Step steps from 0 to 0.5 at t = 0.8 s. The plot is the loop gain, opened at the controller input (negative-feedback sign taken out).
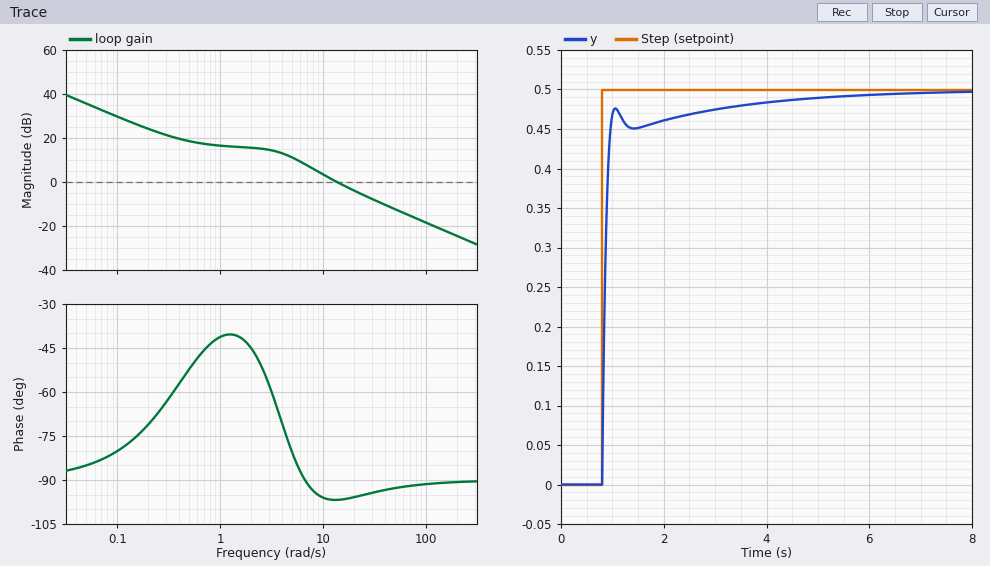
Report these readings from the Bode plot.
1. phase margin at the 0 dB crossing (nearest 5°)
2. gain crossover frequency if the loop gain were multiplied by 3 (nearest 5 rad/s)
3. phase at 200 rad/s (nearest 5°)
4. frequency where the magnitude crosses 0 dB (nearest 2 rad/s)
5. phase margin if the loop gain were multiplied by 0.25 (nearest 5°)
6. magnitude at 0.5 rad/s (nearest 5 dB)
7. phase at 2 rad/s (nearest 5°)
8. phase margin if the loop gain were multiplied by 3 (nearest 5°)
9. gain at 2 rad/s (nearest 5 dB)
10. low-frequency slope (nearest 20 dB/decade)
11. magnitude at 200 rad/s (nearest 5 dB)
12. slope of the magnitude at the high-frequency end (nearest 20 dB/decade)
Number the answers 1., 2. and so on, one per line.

1. 85°
2. 35 rad/s
3. -90°
4. 14 rad/s
5. 105°
6. 20 dB
7. -45°
8. 85°
9. 15 dB
10. -20 dB/decade
11. -25 dB
12. -20 dB/decade
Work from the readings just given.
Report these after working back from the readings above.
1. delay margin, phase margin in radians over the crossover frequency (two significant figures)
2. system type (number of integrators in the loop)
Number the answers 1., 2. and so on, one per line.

1. 0.11 s
2. 1
